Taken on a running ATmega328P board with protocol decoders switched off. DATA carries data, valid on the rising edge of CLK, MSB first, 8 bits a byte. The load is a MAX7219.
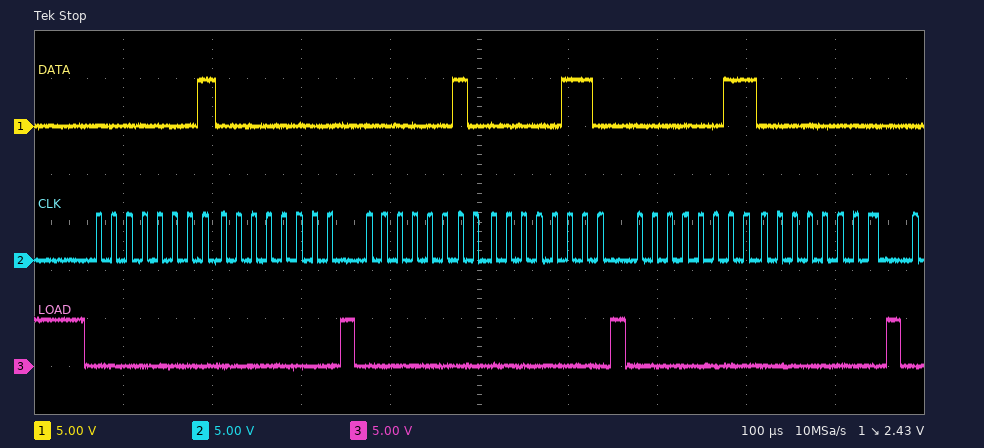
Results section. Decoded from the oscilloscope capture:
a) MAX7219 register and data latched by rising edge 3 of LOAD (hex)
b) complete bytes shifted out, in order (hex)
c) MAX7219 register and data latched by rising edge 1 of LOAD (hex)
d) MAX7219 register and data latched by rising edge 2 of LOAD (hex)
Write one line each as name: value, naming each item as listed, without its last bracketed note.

MAX7219 register and data latched by rising edge 3 of LOAD: register 0x3, data 0x00
complete bytes shifted out, in order: 01 00 02 06 03 00
MAX7219 register and data latched by rising edge 1 of LOAD: register 0x1, data 0x00
MAX7219 register and data latched by rising edge 2 of LOAD: register 0x2, data 0x06
